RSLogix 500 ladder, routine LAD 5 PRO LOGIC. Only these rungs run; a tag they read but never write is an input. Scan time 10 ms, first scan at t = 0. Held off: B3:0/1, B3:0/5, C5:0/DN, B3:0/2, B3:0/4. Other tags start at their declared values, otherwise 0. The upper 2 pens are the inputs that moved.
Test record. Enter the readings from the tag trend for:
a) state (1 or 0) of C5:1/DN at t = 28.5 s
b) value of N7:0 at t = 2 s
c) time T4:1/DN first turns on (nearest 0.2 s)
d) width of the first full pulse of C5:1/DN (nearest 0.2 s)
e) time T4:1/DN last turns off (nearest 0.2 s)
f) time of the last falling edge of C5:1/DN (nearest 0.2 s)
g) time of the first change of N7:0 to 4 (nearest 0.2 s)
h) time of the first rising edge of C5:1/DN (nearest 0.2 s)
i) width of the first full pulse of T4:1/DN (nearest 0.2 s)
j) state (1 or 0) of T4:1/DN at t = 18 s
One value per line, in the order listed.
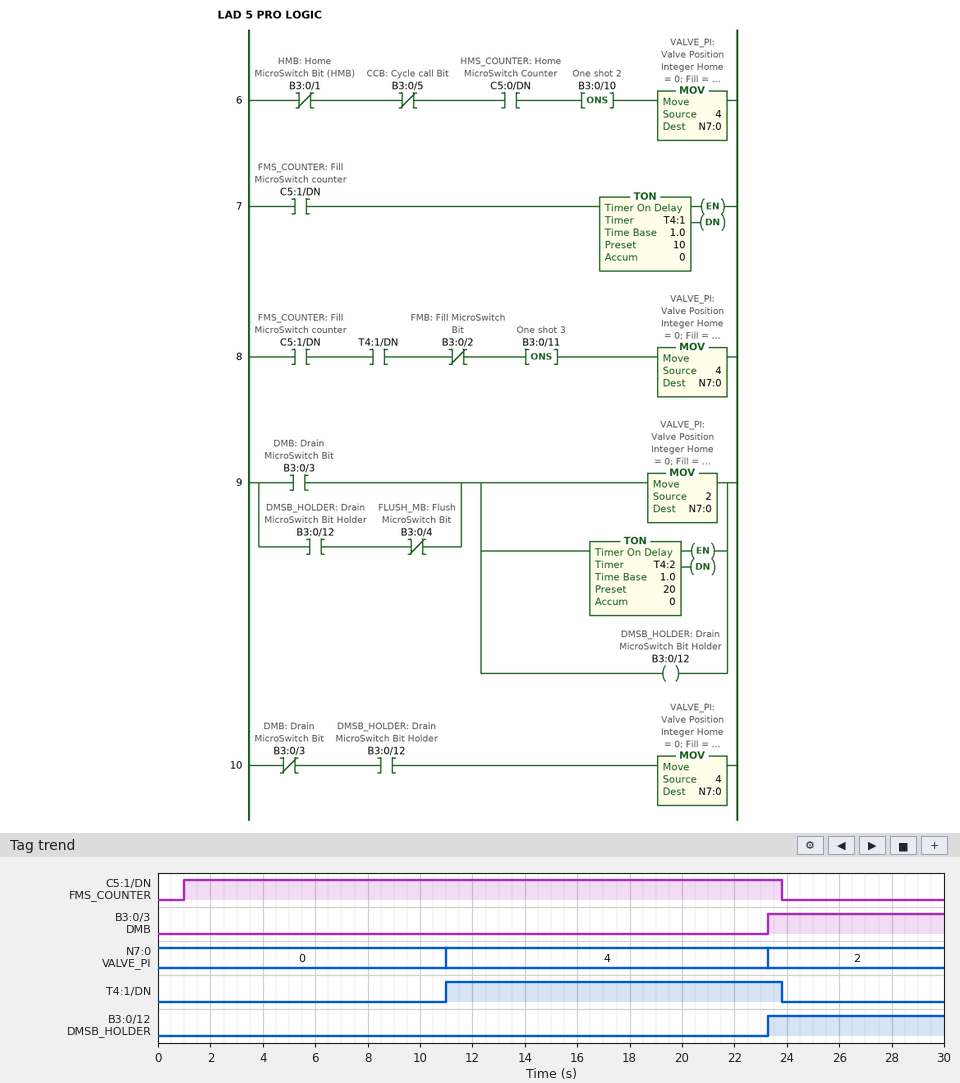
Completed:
0
0
11.0 s
22.8 s
23.8 s
23.8 s
11.0 s
1.0 s
12.8 s
1
